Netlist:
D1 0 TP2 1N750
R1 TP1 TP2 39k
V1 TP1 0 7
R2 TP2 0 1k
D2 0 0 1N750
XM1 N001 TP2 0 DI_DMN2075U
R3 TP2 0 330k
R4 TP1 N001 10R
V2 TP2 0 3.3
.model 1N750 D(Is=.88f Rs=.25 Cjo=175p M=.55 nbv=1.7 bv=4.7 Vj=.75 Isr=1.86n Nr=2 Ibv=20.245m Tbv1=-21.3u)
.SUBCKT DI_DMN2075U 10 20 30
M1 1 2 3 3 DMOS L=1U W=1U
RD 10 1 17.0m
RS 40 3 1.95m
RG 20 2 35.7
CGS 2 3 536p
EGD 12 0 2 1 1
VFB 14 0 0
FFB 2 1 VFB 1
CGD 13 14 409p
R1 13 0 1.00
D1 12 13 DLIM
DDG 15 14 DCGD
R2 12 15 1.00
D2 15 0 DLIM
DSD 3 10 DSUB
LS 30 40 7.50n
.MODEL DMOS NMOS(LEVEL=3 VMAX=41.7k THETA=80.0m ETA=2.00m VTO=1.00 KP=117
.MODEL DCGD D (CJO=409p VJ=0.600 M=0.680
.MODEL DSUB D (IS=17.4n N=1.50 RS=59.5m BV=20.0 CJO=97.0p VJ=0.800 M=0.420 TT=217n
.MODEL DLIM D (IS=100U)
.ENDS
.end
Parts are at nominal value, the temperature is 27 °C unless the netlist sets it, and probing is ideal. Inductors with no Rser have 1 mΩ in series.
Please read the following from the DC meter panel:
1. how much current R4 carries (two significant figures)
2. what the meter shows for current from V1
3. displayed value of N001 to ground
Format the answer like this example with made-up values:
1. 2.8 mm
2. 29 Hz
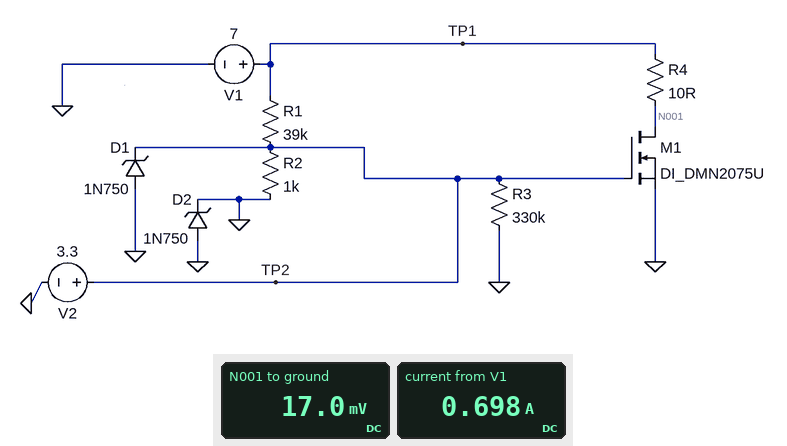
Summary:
1. 700 mA
2. 0.698 A
3. 17.0 mV
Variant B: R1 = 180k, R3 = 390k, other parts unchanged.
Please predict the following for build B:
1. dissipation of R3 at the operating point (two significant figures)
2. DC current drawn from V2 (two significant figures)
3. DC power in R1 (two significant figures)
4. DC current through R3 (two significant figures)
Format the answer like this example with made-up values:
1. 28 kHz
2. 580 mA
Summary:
1. 28 µW
2. 3.3 mA
3. 76 µW
4. 8.5 µA
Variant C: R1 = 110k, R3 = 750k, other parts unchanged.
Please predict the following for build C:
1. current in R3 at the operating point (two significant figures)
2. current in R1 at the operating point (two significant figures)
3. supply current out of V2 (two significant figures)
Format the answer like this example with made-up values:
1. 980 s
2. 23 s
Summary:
1. 4.4 µA
2. 34 µA
3. 3.3 mA
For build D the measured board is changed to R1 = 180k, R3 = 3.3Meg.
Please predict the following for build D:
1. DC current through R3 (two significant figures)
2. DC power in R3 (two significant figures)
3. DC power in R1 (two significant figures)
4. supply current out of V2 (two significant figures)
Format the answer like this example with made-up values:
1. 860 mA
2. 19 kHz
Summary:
1. 1.0 µA
2. 3.3 µW
3. 76 µW
4. 3.3 mA
